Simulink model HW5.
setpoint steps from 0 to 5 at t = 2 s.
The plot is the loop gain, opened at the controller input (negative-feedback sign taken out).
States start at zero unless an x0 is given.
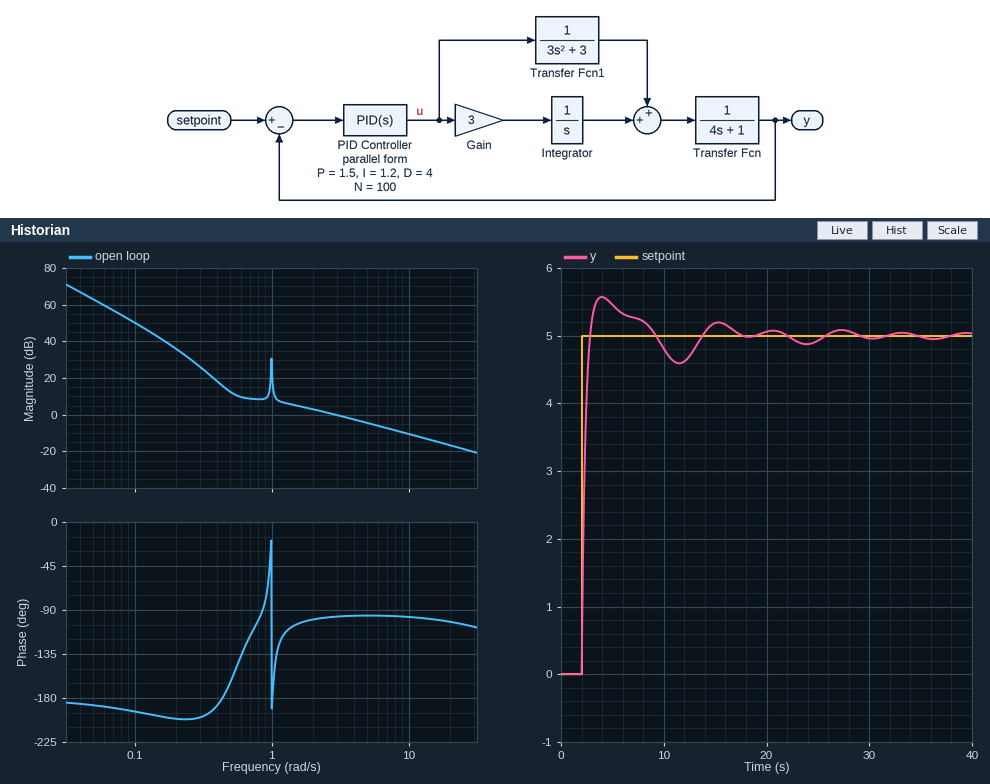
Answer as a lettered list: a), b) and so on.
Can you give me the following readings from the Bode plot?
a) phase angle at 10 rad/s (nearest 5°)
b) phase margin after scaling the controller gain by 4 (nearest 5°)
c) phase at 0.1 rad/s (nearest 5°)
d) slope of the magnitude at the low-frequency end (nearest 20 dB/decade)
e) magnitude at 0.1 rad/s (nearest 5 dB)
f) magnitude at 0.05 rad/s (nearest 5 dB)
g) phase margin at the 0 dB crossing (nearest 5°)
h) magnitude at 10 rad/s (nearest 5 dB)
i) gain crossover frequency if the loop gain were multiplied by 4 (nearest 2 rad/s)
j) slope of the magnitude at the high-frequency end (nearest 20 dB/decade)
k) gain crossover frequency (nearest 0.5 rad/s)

a) -95°
b) 80°
c) -195°
d) -40 dB/decade
e) 50 dB
f) 65 dB
g) 85°
h) -10 dB
i) 12 rad/s
j) -20 dB/decade
k) 3.0 rad/s
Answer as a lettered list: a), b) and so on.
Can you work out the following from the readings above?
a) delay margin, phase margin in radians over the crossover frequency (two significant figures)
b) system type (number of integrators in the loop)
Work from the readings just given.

a) 0.49 s
b) 2
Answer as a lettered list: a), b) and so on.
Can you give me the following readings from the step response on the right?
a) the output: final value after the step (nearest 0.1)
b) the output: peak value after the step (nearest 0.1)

a) 5.0
b) 5.6
